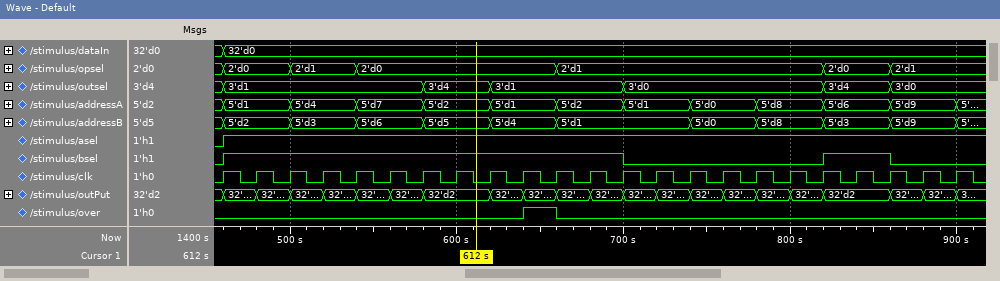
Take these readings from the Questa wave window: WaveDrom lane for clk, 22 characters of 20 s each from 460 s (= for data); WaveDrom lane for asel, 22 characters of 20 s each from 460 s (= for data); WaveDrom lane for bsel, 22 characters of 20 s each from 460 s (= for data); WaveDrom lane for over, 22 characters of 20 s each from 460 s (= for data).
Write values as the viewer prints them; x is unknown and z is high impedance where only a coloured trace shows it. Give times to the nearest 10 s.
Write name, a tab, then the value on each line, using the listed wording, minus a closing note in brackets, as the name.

WaveDrom lane for clk, 22 characters of 20 s each from 460 s	{name: 'clk', wave: 'p.....................'}
WaveDrom lane for asel, 22 characters of 20 s each from 460 s	{name: 'asel', wave: '1.....................'}
WaveDrom lane for bsel, 22 characters of 20 s each from 460 s	{name: 'bsel', wave: '1...........0.....1.0.'}
WaveDrom lane for over, 22 characters of 20 s each from 460 s	{name: 'over', wave: '0........10...........'}
